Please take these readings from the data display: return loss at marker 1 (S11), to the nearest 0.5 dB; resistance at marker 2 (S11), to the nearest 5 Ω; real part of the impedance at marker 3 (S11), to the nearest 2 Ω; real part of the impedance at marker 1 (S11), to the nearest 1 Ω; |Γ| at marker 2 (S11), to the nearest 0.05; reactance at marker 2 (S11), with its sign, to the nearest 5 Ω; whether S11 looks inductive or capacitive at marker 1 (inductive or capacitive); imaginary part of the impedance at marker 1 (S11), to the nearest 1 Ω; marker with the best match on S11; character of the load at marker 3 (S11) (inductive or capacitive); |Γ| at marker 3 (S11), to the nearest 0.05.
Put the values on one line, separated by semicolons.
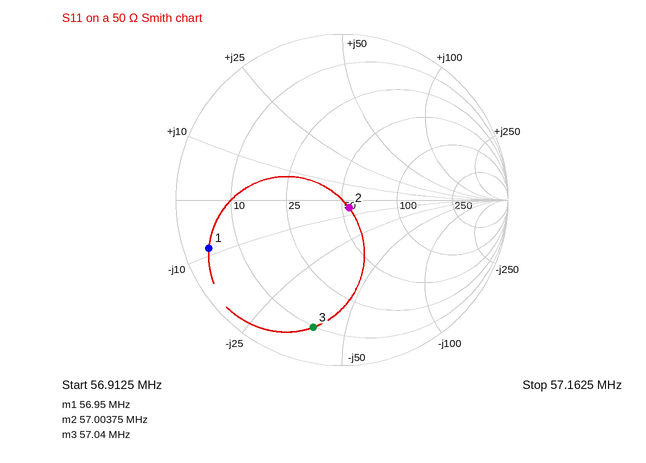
1.5 dB; 55 Ω; 10 Ω; 4 Ω; 0.05; -5 Ω; capacitive; -9 Ω; marker 2; capacitive; 0.80
